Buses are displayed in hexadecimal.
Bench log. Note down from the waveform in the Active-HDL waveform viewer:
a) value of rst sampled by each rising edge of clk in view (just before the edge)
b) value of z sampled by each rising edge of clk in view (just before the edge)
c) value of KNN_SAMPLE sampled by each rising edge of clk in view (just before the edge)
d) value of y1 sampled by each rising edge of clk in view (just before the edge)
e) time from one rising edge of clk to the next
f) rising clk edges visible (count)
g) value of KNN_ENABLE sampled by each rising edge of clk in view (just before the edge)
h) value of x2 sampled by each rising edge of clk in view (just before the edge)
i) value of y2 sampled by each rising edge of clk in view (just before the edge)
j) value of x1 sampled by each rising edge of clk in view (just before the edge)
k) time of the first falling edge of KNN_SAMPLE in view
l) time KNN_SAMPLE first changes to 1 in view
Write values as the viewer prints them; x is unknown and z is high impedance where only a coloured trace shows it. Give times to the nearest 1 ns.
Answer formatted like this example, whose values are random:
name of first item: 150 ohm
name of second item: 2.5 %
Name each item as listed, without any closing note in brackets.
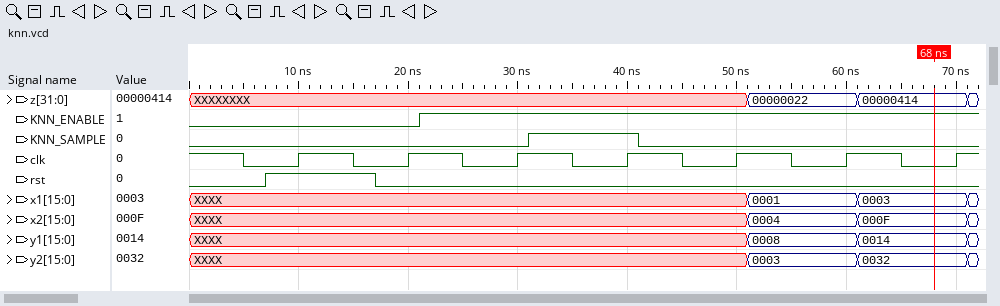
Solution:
value of rst sampled by each rising edge of clk in view: 1 0 0 0 0 0 0
value of z sampled by each rising edge of clk in view: XXXXXXXX, XXXXXXXX, XXXXXXXX, XXXXXXXX, XXXXXXXX, 00000022, 00000414
value of KNN_SAMPLE sampled by each rising edge of clk in view: 0 0 0 1 0 0 0
value of y1 sampled by each rising edge of clk in view: XXXX, XXXX, XXXX, XXXX, XXXX, 0008, 0014
time from one rising edge of clk to the next: 10 ns
rising clk edges visible: 7
value of KNN_ENABLE sampled by each rising edge of clk in view: 0 0 1 1 1 1 1
value of x2 sampled by each rising edge of clk in view: XXXX, XXXX, XXXX, XXXX, XXXX, 0004, 000F
value of y2 sampled by each rising edge of clk in view: XXXX, XXXX, XXXX, XXXX, XXXX, 0003, 0032
value of x1 sampled by each rising edge of clk in view: XXXX, XXXX, XXXX, XXXX, XXXX, 0001, 0003
time of the first falling edge of KNN_SAMPLE in view: 41 ns
time KNN_SAMPLE first changes to 1 in view: 31 ns
